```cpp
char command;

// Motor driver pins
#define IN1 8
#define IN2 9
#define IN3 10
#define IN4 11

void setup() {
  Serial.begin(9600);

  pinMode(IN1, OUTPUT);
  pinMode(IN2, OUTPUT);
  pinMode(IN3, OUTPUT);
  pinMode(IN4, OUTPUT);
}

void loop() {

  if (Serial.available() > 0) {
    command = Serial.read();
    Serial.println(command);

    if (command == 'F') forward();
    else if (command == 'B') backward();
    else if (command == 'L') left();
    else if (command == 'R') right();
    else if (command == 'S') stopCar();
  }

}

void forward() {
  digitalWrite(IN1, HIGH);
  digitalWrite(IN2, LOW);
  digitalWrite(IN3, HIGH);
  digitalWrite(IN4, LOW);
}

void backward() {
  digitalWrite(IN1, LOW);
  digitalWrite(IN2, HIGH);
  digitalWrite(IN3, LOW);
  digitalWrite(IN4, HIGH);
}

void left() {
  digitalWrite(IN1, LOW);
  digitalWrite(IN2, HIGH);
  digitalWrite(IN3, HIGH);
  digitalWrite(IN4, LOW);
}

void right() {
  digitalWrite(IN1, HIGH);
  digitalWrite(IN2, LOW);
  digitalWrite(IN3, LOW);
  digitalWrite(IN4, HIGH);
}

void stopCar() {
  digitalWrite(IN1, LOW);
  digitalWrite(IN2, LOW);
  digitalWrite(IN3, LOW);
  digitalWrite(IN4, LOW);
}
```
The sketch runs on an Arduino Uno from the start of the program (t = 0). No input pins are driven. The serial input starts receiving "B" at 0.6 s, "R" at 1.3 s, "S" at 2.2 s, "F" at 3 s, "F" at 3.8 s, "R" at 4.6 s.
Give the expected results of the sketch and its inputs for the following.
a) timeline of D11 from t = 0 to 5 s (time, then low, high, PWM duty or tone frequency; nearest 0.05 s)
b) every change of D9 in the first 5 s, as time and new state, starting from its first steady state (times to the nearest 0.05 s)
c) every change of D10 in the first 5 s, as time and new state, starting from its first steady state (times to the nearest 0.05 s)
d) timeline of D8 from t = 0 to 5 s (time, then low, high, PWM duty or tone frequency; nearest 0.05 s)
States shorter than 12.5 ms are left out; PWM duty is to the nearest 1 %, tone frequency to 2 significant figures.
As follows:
0 s low; 0.6 s high; 2.2 s low; 4.6 s high
0 s low; 0.6 s high; 1.3 s low
0 s low; 3 s high; 4.6 s low
0 s low; 1.3 s high; 2.2 s low; 3 s high
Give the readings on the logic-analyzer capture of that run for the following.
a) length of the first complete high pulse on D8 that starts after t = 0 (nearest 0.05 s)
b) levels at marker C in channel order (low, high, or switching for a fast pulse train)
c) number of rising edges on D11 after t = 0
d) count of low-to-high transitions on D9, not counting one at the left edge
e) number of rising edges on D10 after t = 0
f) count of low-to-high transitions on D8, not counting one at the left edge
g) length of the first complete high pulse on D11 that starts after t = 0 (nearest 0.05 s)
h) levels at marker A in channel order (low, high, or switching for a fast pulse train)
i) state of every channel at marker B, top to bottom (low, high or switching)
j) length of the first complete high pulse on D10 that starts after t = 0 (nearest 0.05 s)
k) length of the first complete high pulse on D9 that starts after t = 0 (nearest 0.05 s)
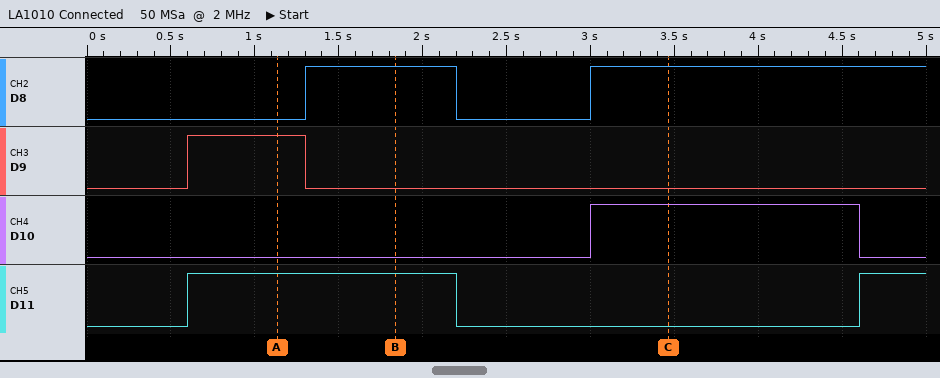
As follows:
0.90 s
D8 high, D9 low, D10 high, D11 low
2
1
1
2
1.60 s
D8 low, D9 high, D10 low, D11 high
D8 high, D9 low, D10 low, D11 high
1.60 s
0.70 s
